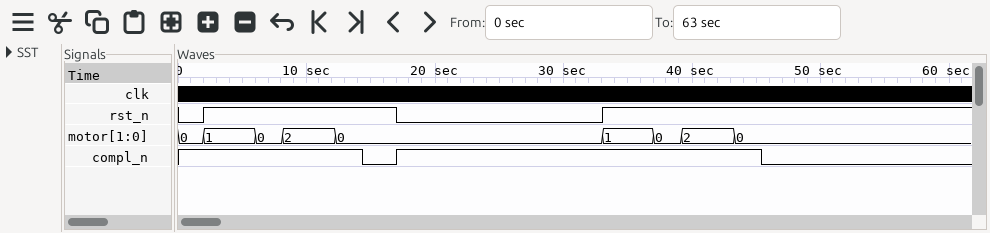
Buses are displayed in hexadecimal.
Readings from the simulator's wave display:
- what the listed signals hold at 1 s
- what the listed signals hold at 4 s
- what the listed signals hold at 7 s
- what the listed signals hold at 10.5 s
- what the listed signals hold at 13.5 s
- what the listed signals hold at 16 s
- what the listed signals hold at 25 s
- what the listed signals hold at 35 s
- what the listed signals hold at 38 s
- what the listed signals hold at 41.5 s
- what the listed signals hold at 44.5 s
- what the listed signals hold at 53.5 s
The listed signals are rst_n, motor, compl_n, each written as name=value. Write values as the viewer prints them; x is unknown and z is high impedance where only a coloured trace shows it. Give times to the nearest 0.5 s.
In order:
rst_n=0, motor=0, compl_n=1
rst_n=1, motor=1, compl_n=1
rst_n=1, motor=0, compl_n=1
rst_n=1, motor=2, compl_n=1
rst_n=1, motor=0, compl_n=1
rst_n=1, motor=0, compl_n=0
rst_n=0, motor=0, compl_n=1
rst_n=1, motor=1, compl_n=1
rst_n=1, motor=0, compl_n=1
rst_n=1, motor=2, compl_n=1
rst_n=1, motor=0, compl_n=1
rst_n=1, motor=0, compl_n=0
